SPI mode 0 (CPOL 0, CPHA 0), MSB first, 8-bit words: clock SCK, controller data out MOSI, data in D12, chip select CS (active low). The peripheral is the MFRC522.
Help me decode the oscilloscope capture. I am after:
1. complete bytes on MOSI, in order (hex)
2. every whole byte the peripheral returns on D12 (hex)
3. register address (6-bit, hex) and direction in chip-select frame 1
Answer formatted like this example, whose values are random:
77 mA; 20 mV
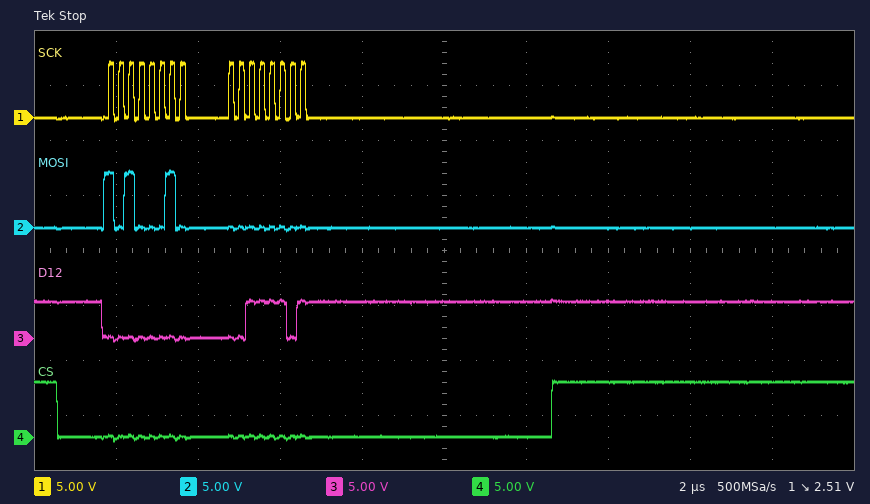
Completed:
0xA2 0x00; 0x00 0x3D; 0x11 read
